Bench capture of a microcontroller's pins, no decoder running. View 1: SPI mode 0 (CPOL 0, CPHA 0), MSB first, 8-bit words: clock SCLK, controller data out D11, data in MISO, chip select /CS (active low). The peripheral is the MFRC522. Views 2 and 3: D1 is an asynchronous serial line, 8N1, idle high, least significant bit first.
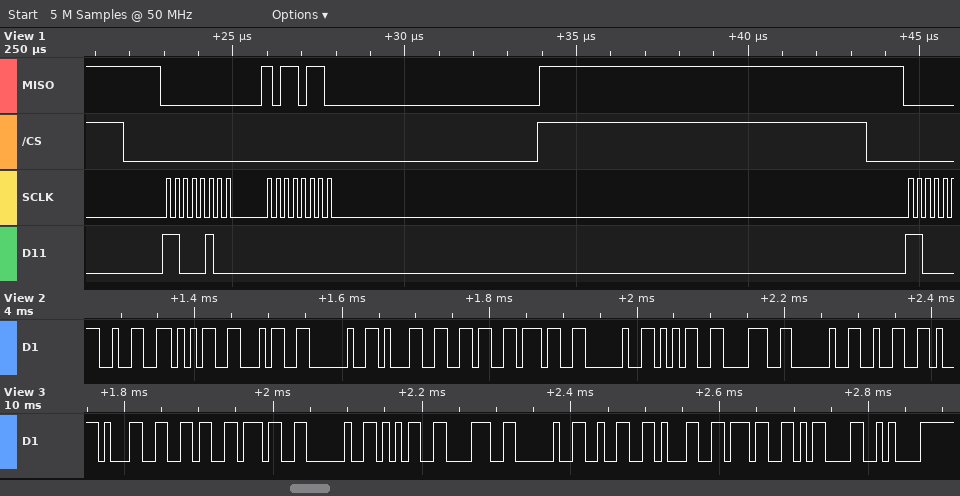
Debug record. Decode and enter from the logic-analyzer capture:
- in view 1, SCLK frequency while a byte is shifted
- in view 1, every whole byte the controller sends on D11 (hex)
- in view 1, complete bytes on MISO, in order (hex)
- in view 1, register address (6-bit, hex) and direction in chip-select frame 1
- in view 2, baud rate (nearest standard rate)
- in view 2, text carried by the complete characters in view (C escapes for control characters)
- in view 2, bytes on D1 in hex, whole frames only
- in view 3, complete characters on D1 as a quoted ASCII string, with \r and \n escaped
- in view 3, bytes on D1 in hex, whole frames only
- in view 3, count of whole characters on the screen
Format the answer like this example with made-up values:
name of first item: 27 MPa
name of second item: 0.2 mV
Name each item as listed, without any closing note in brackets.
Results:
in view 1, SCLK frequency while a byte is shifted: 4 MHz
in view 1, every whole byte the controller sends on D11: C4 00
in view 1, complete bytes on MISO, in order: 00 B6
in view 1, register address (6-bit, hex) and direction in chip-select frame 1: 0x22 read
in view 2, baud rate: 115200 baud
in view 2, text carried by the complete characters in view: "254 167 58 2"
in view 2, bytes on D1 in hex, whole frames only: 32 35 34 20 31 36 37 20 35 38 20 32
in view 3, complete characters on D1 as a quoted ASCII string, with \r and \n escaped: "167 58 217\r\n"
in view 3, bytes on D1 in hex, whole frames only: 0x31 0x36 0x37 0x20 0x35 0x38 0x20 0x32 0x31 0x37 0x0D 0x0A
in view 3, count of whole characters on the screen: 12
